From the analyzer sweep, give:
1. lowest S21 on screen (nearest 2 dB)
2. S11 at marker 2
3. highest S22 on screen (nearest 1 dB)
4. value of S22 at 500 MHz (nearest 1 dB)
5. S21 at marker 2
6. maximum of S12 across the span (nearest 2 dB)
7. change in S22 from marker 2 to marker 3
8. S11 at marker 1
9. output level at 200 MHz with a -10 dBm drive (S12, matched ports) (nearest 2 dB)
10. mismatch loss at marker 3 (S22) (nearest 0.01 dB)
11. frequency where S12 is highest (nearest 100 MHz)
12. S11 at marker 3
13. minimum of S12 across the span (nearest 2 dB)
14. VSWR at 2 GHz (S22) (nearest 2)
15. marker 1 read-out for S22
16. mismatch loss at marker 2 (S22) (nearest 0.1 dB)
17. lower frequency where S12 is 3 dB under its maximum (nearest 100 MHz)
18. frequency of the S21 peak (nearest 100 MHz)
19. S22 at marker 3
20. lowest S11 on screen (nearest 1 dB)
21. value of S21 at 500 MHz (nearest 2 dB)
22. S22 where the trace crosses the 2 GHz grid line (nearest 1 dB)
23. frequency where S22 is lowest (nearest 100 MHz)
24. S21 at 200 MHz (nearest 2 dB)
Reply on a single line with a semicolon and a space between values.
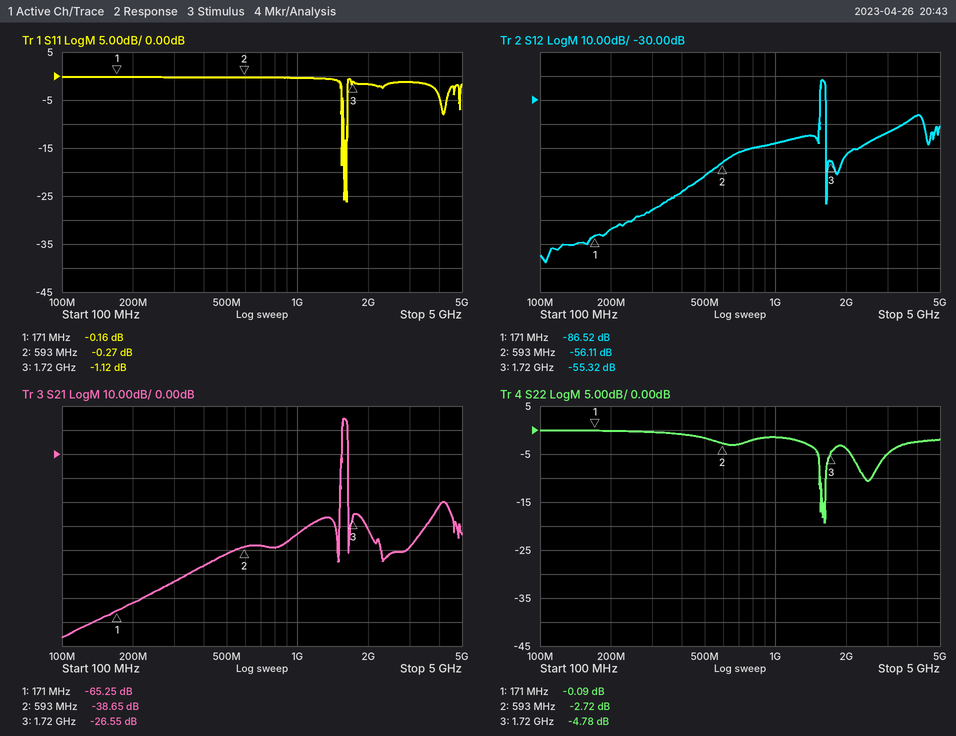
-76 dB; -0.27 dB; 0 dB; -2 dB; -38.65 dB; -22 dB; -2.06 dB; -0.16 dB; -94 dBm; 1.76 dB; 1.6 GHz; -1.12 dB; -98 dB; 4; -0.09 dB; 3.3 dB; 1.6 GHz; 1.6 GHz; -4.78 dB; -26 dB; -42 dB; -4 dB; 1.6 GHz; -62 dB
